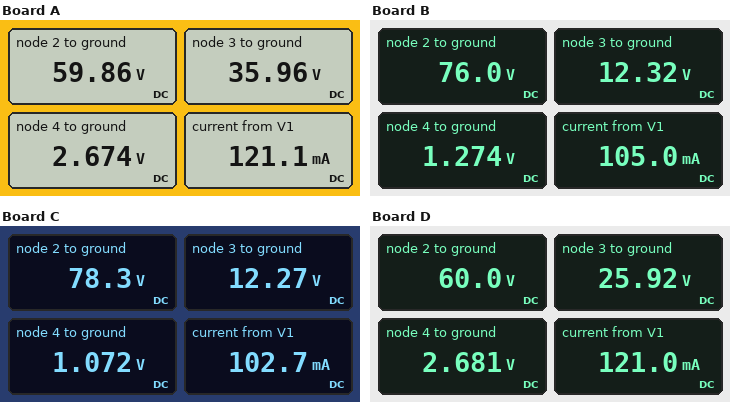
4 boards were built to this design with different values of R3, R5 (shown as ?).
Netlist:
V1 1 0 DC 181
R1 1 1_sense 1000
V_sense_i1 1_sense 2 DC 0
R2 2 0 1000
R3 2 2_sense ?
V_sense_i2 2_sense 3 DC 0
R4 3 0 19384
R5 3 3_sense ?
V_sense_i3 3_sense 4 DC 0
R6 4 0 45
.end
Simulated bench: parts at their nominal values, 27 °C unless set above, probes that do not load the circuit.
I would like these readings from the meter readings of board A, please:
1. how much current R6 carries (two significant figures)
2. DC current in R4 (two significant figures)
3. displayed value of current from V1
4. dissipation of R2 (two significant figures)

59 mA
1.9 mA
121.1 mA
3.6 W
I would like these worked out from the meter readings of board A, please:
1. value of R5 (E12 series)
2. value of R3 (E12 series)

560 Ω
390 Ω
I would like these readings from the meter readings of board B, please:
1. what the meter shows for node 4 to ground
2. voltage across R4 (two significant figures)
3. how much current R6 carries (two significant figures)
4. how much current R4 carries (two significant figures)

1.274 V
12 V
28 mA
640 µA
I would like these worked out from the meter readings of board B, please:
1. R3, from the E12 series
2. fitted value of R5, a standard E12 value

2.2 kΩ
390 Ω
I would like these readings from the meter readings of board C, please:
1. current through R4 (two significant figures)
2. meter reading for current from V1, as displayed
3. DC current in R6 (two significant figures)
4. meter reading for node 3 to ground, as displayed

630 µA
102.7 mA
24 mA
12.27 V
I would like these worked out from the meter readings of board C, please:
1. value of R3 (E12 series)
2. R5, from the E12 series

2.7 kΩ
470 Ω
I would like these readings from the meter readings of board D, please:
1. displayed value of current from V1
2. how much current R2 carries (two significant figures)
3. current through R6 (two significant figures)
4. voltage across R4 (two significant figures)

121.0 mA
60 mA
60 mA
26 V
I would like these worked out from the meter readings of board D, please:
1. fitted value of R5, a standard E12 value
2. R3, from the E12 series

390 Ω
560 Ω
